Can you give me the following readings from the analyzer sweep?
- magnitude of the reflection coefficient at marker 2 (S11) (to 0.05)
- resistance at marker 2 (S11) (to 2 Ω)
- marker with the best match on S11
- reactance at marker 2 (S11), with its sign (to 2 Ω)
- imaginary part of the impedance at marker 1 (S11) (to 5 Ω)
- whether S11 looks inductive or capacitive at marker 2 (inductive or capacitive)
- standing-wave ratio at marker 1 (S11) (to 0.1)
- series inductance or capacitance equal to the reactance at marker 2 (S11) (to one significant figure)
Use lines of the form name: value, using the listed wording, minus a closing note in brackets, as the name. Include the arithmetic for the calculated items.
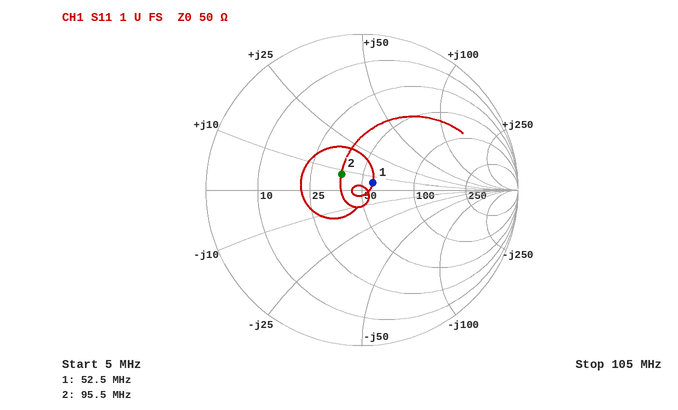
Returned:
magnitude of the reflection coefficient at marker 2 (S11): 0.15
resistance at marker 2 (S11): 38 Ω
marker with the best match on S11: marker 1
reactance at marker 2 (S11), with its sign: +8 Ω
imaginary part of the impedance at marker 1 (S11): +5 Ω
whether S11 looks inductive or capacitive at marker 2: inductive
standing-wave ratio at marker 1 (S11): 1.2
series inductance or capacitance equal to the reactance at marker 2 (S11): L = 8 Ω/(2π × 95.5 MHz) ≈ 13.3 nH, so 10 nH to one significant figure
